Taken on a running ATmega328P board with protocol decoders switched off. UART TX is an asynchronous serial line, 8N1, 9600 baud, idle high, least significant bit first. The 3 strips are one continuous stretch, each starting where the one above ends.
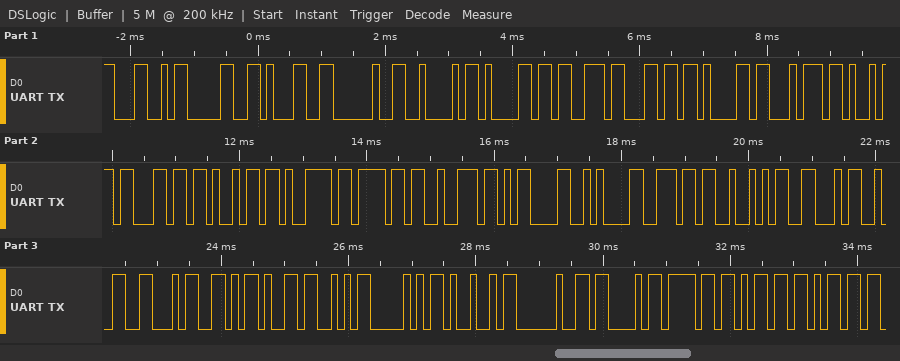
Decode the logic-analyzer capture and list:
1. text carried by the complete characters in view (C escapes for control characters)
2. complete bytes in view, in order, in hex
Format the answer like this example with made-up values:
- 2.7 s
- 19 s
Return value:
- "L01 Baslatiliyor\r\nnRF24-SPI Comm"
- 0x4C 0x30 0x31 0x20 0x42 0x61 0x73 0x6C 0x61 0x74 0x69 0x6C 0x69 0x79 0x6F 0x72 0x0D 0x0A 0x6E 0x52 0x46 0x32 0x34 0x2D 0x53 0x50 0x49 0x20 0x43 0x6F 0x6D 0x6D
